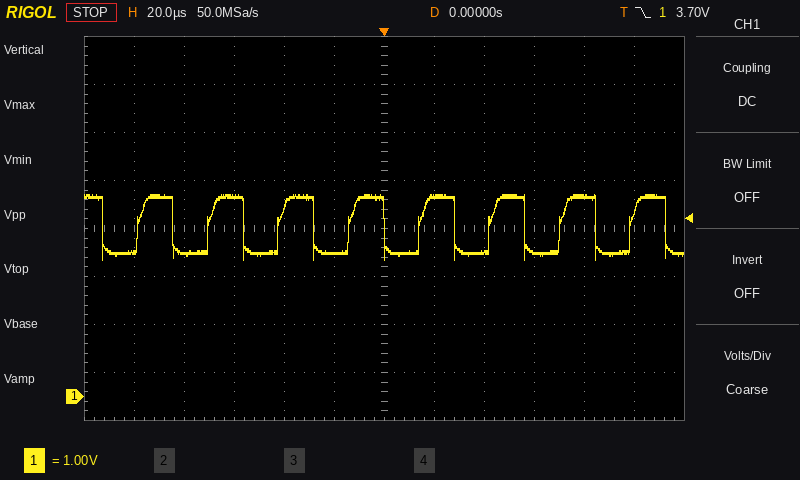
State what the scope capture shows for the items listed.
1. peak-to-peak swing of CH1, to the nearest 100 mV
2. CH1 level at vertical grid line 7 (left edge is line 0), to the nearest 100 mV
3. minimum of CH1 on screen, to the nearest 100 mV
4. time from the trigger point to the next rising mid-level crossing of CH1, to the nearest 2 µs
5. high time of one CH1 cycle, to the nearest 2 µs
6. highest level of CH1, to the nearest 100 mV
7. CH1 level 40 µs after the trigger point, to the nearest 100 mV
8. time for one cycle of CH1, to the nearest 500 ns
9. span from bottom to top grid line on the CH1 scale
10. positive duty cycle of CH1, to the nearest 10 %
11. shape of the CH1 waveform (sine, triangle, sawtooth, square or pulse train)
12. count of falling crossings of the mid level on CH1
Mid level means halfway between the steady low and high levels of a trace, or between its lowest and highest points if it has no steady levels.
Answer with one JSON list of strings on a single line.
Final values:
["1.4 V", "4.2 V", "2.8 V", "14 µs", "14 µs", "4.2 V", "3.0 V", "28.0 µs", "8 V", "50 %", "square", "9"]
